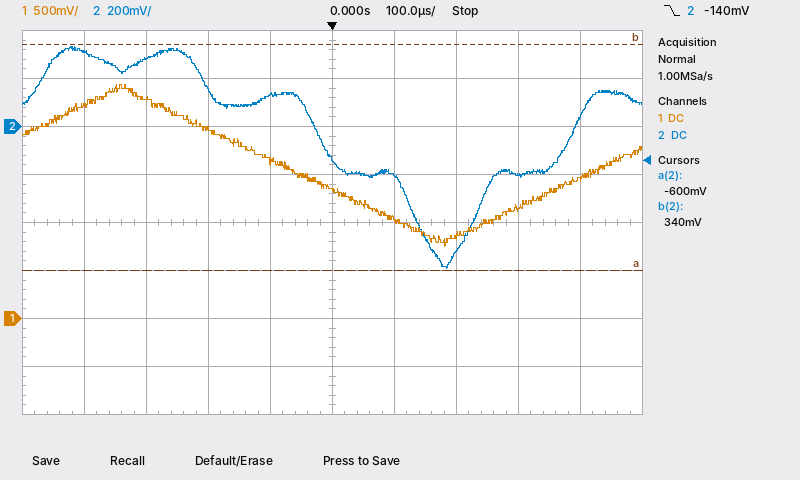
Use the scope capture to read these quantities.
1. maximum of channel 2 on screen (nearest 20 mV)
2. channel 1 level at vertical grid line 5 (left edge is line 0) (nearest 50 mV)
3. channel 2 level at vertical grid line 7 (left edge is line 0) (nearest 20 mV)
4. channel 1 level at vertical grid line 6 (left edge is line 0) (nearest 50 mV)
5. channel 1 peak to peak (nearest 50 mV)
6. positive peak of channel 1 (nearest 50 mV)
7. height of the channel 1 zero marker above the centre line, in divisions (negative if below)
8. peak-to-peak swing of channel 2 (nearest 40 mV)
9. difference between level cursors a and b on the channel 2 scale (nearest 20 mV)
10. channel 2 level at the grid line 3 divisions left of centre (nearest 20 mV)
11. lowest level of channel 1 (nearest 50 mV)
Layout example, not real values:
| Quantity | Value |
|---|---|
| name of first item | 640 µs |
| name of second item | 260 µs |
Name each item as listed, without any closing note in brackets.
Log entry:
| Quantity | Value |
|---|---|
| maximum of channel 2 on screen | 340 mV |
| channel 1 level at vertical grid line 5 (left edge is line 0) | 1.35 V |
| channel 2 level at vertical grid line 7 (left edge is line 0) | -520 mV |
| channel 1 level at vertical grid line 6 (left edge is line 0) | 1.05 V |
| channel 1 peak to peak | 1.70 V |
| positive peak of channel 1 | 2.45 V |
| height of the channel 1 zero marker above the centre line, in divisions | -2.0 div |
| peak-to-peak swing of channel 2 | 920 mV |
| difference between level cursors a and b on the channel 2 scale | 940 mV |
| channel 2 level at the grid line 3 divisions left of centre | 280 mV |
| lowest level of channel 1 | 750 mV |
